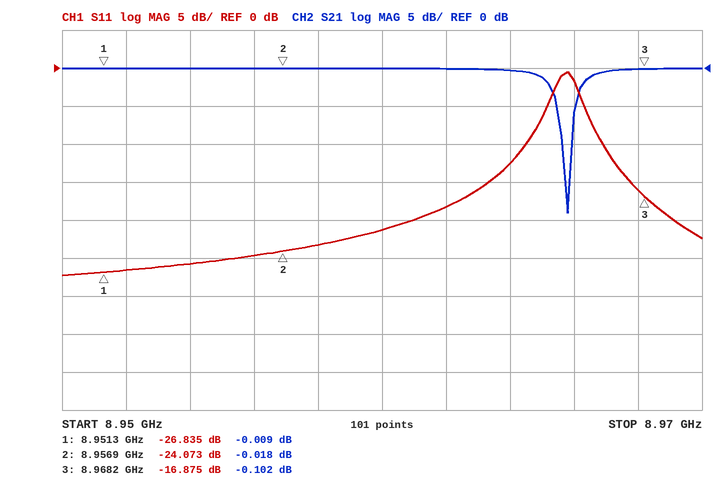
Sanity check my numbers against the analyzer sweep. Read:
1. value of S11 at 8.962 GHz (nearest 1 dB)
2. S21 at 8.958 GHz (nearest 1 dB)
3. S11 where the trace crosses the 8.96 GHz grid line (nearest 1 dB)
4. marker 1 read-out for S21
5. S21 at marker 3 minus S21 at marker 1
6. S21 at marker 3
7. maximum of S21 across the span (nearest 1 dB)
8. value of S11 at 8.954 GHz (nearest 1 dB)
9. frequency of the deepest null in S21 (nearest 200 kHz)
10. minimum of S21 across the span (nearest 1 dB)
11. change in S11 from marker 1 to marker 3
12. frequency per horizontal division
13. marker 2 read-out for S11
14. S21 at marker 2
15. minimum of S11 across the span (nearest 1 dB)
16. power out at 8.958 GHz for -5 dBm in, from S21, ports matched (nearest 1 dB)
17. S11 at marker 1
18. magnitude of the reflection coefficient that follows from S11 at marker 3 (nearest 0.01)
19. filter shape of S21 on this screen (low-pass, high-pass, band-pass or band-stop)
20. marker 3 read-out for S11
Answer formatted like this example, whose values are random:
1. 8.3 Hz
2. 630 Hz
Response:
1. -18 dB
2. 0 dB
3. -21 dB
4. -0.009 dB
5. -0.093 dB
6. -0.102 dB
7. 0 dB
8. -26 dB
9. 8.9658 GHz
10. -19 dB
11. 9.960 dB
12. 2 MHz
13. -24.073 dB
14. -0.018 dB
15. -27 dB
16. -5 dBm
17. -26.835 dB
18. 0.14
19. band-stop
20. -16.875 dB
